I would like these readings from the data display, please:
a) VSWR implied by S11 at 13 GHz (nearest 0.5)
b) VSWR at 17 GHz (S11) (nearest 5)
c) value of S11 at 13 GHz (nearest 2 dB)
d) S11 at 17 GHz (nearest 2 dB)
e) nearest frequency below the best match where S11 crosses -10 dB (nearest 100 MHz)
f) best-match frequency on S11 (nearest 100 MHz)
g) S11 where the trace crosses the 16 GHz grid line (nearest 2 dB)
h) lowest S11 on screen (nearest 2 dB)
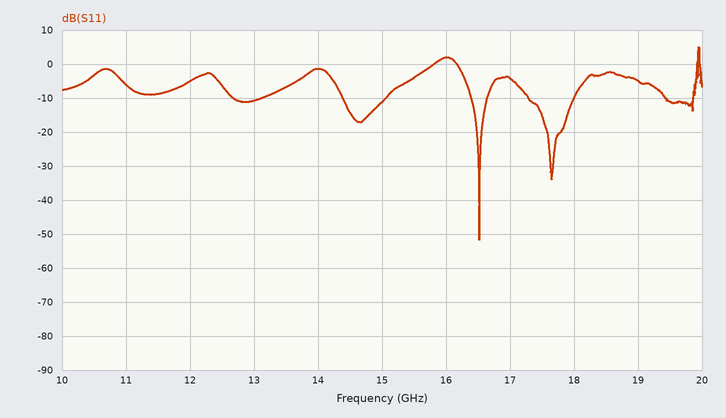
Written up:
2.0
5
-10 dB
-4 dB
16.4 GHz
16.5 GHz
2 dB
-52 dB
